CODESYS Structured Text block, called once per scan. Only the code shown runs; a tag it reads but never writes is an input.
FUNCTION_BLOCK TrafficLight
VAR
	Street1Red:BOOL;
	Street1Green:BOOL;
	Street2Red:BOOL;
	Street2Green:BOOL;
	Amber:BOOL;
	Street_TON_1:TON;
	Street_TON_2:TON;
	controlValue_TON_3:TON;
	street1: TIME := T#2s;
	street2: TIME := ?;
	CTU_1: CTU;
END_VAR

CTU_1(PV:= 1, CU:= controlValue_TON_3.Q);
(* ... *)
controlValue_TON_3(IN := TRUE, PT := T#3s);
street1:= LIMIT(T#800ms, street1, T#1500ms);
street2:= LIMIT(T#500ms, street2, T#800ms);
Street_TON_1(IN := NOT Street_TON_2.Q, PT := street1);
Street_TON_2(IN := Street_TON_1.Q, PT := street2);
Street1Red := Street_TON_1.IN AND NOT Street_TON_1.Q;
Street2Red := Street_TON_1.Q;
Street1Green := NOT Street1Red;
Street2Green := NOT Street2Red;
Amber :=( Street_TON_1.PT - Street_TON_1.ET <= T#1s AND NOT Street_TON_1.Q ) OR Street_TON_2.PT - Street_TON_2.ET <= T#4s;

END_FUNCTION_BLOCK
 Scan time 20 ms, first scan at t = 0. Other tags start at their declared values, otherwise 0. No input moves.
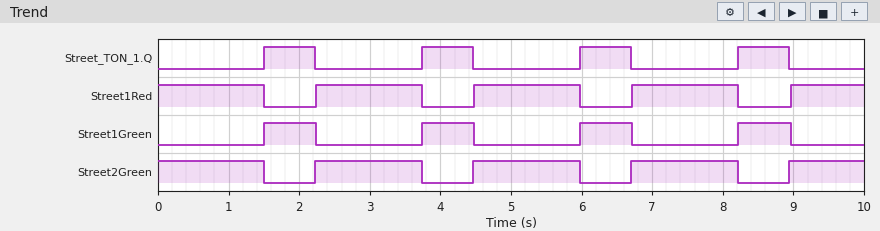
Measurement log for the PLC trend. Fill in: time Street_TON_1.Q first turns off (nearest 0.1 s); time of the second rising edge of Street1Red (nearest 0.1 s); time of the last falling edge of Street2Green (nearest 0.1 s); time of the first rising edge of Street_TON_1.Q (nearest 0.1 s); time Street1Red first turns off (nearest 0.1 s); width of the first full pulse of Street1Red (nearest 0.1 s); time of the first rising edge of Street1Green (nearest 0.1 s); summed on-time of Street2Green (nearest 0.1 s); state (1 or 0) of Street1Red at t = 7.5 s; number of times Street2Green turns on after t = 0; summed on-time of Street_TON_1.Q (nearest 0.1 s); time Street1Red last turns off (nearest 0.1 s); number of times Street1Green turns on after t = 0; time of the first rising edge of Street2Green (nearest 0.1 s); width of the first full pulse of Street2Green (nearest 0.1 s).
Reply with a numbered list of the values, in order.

1. 2.2 s
2. 4.5 s
3. 8.2 s
4. 1.5 s
5. 1.5 s
6. 1.5 s
7. 1.5 s
8. 7.1 s
9. 1
10. 4
11. 2.9 s
12. 8.2 s
13. 4
14. 2.2 s
15. 1.5 s
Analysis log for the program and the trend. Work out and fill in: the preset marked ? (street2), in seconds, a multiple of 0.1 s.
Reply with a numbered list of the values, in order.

1. 0.7 s
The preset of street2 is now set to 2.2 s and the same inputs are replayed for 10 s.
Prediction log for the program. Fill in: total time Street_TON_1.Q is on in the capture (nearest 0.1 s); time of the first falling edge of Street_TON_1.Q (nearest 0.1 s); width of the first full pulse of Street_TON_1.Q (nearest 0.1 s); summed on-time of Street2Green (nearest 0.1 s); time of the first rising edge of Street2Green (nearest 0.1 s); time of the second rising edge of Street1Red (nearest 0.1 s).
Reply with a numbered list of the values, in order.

1. 3.3 s
2. 2.3 s
3. 0.8 s
4. 6.7 s
5. 2.3 s
6. 4.7 s
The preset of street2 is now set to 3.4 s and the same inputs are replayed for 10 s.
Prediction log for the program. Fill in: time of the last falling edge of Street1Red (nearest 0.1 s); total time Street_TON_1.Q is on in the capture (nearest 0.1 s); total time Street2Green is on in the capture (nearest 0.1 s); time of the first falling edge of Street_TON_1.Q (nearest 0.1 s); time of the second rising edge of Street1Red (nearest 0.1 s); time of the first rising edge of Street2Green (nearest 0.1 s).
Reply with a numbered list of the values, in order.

1. 8.5 s
2. 3.3 s
3. 6.7 s
4. 2.3 s
5. 4.7 s
6. 2.3 s
